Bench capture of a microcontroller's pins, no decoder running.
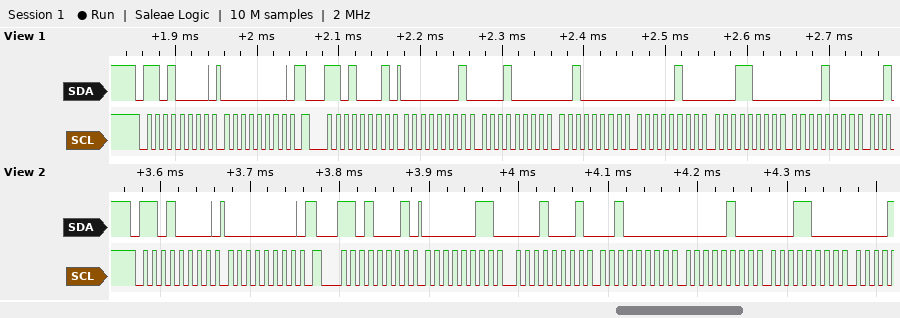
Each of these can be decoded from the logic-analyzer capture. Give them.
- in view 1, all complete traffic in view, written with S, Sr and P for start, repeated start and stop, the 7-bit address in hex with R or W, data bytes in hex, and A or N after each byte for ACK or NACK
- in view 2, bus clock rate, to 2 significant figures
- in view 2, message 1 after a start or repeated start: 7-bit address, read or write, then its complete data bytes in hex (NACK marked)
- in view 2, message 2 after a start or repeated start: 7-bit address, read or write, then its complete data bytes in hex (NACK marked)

S 68W A 00 A Sr 68R A 01 A 10 A 20 A 04 A 18 A 08 A
100 kHz
0x68 write: 00
0x68 read: 03 11 20 04 18
